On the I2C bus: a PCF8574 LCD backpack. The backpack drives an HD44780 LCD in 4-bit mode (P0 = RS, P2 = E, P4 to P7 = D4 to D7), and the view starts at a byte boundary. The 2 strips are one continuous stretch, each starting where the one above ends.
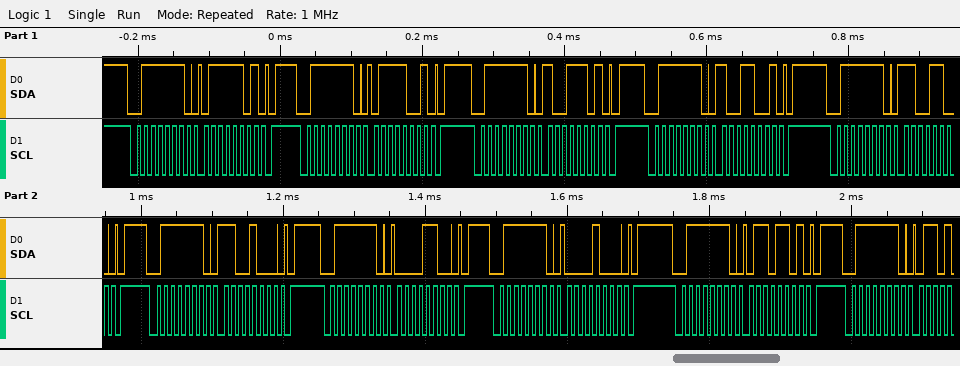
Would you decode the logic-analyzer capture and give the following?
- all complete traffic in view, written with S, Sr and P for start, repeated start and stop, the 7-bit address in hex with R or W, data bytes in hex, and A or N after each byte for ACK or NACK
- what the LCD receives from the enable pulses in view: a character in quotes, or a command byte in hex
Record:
S 3FW A 7D A P S 3FW A 79 A P S 3FW A 9D A P S 3FW A 99 A P S 3FW A CC A P S 3FW A C8 A P S 3FW A 0C A P S 3FW A 08 A P S 3FW A 6D A P S 3FW A
'y' 0xC0
